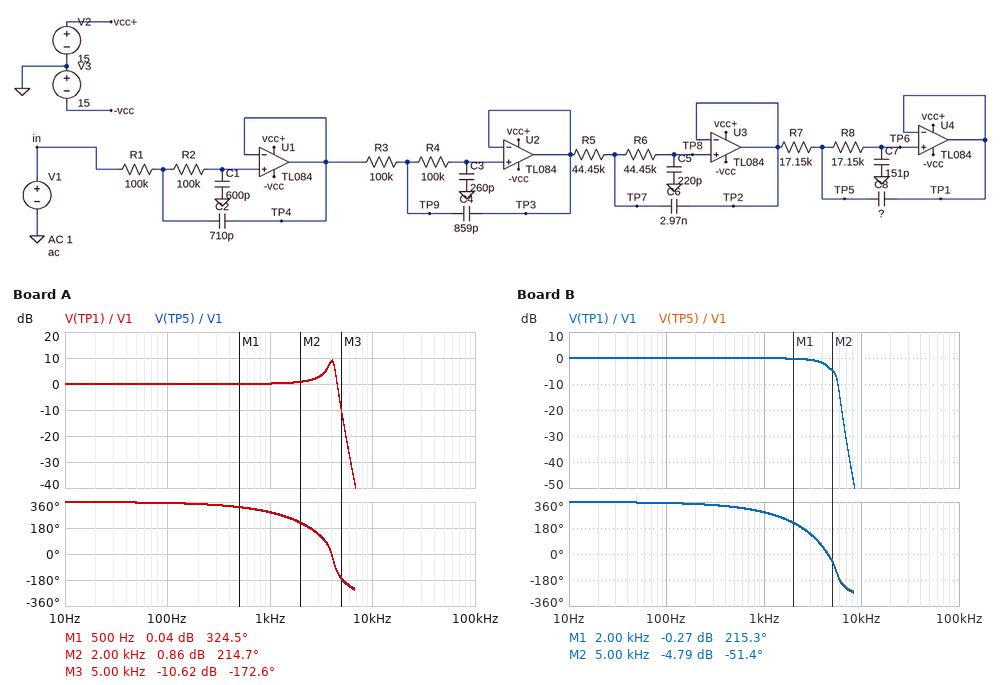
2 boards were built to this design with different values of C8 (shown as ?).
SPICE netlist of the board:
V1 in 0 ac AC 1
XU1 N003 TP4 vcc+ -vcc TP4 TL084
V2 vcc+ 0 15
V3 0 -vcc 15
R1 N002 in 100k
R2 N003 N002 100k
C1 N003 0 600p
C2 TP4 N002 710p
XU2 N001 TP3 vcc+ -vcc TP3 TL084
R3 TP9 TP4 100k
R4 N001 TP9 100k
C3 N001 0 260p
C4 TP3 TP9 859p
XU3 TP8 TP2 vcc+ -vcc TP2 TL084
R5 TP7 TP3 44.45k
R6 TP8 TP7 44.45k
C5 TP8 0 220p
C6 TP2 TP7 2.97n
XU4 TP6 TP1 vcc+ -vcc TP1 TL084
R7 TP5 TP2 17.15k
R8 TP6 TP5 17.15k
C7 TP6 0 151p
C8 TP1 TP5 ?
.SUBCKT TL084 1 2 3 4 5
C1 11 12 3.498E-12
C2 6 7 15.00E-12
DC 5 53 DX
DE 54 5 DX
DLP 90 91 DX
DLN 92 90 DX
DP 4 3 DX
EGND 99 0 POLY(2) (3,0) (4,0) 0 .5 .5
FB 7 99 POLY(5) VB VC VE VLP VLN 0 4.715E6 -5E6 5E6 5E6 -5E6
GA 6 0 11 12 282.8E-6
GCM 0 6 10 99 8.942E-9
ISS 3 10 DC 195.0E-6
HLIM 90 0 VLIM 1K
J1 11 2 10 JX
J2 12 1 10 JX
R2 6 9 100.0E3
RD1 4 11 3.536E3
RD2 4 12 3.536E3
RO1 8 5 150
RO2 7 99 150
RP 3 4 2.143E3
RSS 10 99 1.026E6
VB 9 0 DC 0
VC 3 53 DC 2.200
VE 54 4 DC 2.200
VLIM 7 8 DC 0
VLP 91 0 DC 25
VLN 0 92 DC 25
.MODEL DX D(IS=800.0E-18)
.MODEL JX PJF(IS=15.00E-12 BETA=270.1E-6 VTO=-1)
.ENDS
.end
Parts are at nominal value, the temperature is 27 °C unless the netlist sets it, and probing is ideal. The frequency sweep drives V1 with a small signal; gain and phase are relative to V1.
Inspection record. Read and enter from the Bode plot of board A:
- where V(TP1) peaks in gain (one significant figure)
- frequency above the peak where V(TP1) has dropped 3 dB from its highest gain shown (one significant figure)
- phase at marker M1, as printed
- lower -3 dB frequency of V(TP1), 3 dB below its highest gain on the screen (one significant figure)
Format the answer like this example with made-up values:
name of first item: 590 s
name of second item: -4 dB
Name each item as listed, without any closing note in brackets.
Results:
where V(TP1) peaks in gain: 4 kHz
frequency above the peak where V(TP1) has dropped 3 dB from its highest gain shown: 4 kHz
phase at marker M1, as printed: 324.5 deg
lower -3 dB frequency of V(TP1), 3 dB below its highest gain on the screen: 4 kHz
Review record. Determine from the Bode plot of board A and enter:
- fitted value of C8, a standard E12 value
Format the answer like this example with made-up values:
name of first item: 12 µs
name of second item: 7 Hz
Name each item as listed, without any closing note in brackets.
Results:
fitted value of C8, a standard E12 value: 33 nF
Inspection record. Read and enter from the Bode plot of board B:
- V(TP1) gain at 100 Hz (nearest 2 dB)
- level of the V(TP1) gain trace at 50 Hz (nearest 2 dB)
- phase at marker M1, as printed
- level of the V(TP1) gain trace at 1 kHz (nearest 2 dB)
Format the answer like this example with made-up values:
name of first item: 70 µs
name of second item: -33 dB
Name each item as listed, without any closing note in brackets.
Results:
V(TP1) gain at 100 Hz: 0 dB
level of the V(TP1) gain trace at 50 Hz: 0 dB
phase at marker M1, as printed: 215.3 deg
level of the V(TP1) gain trace at 1 kHz: 0 dB
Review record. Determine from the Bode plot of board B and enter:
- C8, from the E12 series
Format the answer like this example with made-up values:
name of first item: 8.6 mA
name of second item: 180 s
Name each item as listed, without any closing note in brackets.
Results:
C8, from the E12 series: 18 nF
